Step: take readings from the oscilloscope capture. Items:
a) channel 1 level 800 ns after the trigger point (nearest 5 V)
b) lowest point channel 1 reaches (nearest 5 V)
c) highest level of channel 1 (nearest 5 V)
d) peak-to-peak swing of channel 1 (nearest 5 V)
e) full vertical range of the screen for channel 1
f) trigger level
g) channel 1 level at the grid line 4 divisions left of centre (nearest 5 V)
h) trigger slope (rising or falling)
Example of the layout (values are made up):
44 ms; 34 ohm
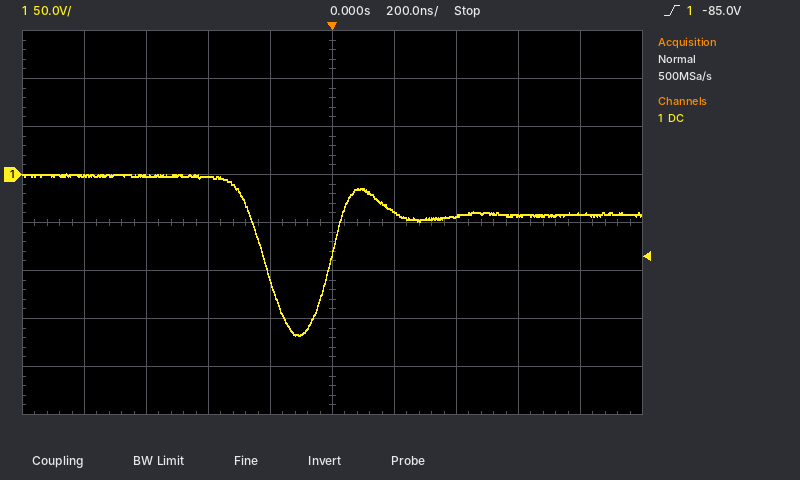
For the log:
-40 V; -170 V; 0 V; 170 V; 400 V; -85.0 V; 0 V; rising
